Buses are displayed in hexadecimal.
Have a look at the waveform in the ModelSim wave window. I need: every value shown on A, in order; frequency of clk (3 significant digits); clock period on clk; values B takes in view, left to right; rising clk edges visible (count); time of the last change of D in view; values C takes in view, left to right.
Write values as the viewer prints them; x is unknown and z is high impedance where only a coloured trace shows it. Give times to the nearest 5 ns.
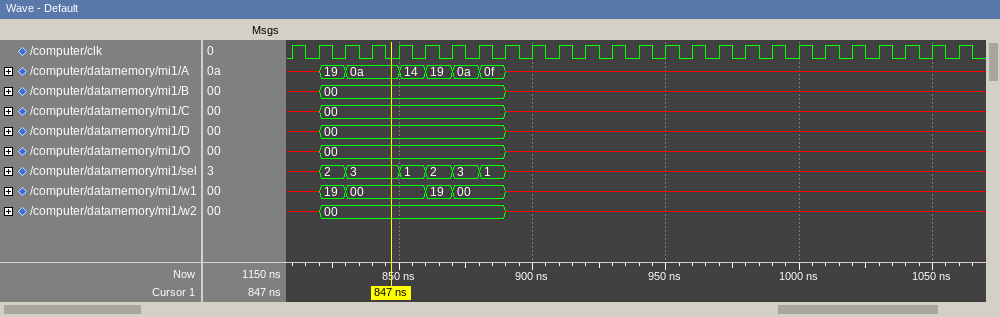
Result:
x, 19, 0a, 14, 19, 0a, 0f, x
100 MHz
10 ns
x, 00, x
26
890 ns
x, 00, x
